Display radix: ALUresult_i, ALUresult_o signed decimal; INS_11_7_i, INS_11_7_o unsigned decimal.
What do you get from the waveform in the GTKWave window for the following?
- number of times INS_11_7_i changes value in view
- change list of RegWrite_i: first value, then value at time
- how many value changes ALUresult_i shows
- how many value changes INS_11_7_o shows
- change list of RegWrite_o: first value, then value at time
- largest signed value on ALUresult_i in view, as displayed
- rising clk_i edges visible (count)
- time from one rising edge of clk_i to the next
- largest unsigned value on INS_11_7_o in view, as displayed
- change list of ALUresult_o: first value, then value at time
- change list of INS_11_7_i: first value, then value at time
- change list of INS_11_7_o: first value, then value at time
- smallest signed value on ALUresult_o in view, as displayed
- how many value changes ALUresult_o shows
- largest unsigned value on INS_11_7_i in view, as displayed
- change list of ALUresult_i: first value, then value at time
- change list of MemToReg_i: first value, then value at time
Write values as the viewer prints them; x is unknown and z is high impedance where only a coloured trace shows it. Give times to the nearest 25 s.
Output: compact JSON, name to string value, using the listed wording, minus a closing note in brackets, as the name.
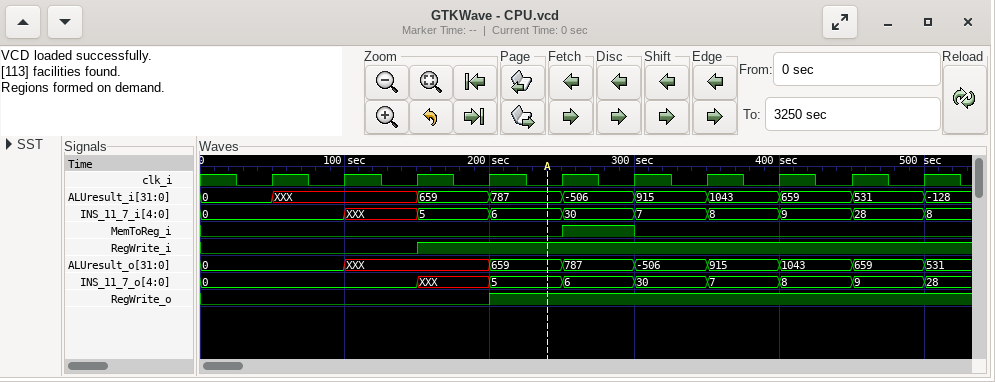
{"number of times INS_11_7_i changes value in view": "9", "change list of RegWrite_i: first value, then value at time": "0, 1 at 150 s", "how many value changes ALUresult_i shows": "9", "how many value changes INS_11_7_o shows": "8", "change list of RegWrite_o: first value, then value at time": "0, 1 at 200 s", "largest signed value on ALUresult_i in view, as displayed": "1043", "rising clk_i edges visible": "10", "time from one rising edge of clk_i to the next": "50 s", "largest unsigned value on INS_11_7_o in view, as displayed": "30", "change list of ALUresult_o: first value, then value at time": "0, XXX at 100 s, 659 at 200 s, 787 at 250 s, -506 at 300 s, 915 at 350 s, 1043 at 400 s, 659 at 450 s, 531 at 500 s", "change list of INS_11_7_i: first value, then value at time": "0, XXX at 100 s, 5 at 150 s, 6 at 200 s, 30 at 250 s, 7 at 300 s, 8 at 350 s, 9 at 400 s, 28 at 450 s, 8 at 500 s", "change list of INS_11_7_o: first value, then value at time": "0, XXX at 150 s, 5 at 200 s, 6 at 250 s, 30 at 300 s, 7 at 350 s, 8 at 400 s, 9 at 450 s, 28 at 500 s", "smallest signed value on ALUresult_o in view, as displayed": "-506", "how many value changes ALUresult_o shows": "8", "largest unsigned value on INS_11_7_i in view, as displayed": "30", "change list of ALUresult_i: first value, then value at time": "0, XXX at 50 s, 659 at 150 s, 787 at 200 s, -506 at 250 s, 915 at 300 s, 1043 at 350 s, 659 at 400 s, 531 at 450 s, -128 at 500 s", "change list of MemToReg_i: first value, then value at time": "0, 1 at 250 s, 0 at 300 s"}
